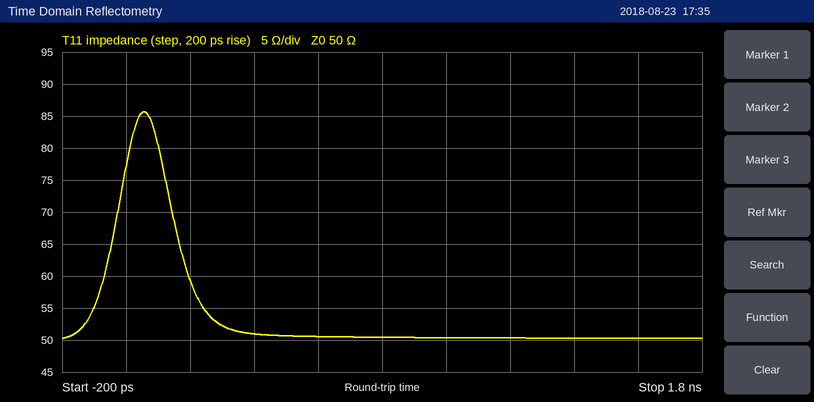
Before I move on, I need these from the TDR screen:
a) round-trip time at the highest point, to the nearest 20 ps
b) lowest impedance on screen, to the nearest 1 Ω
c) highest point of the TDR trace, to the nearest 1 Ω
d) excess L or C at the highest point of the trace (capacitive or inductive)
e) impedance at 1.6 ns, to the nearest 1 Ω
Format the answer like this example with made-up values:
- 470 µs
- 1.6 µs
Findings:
- 60 ps
- 50 Ω
- 86 Ω
- inductive
- 50 Ω
